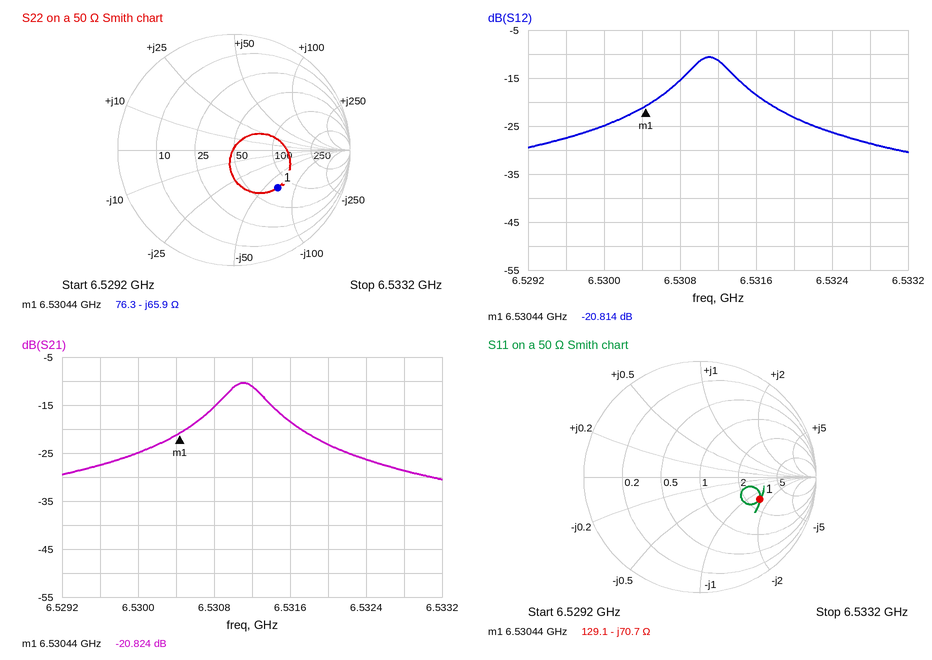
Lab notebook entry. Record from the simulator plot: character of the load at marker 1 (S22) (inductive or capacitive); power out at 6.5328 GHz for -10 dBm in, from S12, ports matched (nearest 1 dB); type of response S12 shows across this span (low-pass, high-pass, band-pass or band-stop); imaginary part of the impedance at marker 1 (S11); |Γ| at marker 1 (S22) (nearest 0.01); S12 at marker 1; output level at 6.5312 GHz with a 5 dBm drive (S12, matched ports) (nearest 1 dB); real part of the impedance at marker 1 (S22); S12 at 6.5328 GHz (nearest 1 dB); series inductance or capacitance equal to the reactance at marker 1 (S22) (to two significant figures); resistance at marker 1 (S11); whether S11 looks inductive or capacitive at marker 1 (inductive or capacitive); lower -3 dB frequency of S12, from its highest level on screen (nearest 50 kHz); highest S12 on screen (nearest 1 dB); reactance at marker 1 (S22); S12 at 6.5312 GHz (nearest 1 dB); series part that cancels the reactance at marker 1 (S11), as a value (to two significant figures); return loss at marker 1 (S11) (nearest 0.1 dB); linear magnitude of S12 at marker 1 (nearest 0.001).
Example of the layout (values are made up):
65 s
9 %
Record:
capacitive
-39 dBm
band-pass
-70.7 Ω
0.50
-20.814 dB
-6 dBm
76.3 Ω
-29 dB
370 fF
129.1 Ω
capacitive
6.53090 GHz
-11 dB
-65.9 Ω
-11 dB
1.7 nH
5.2 dB
0.091
